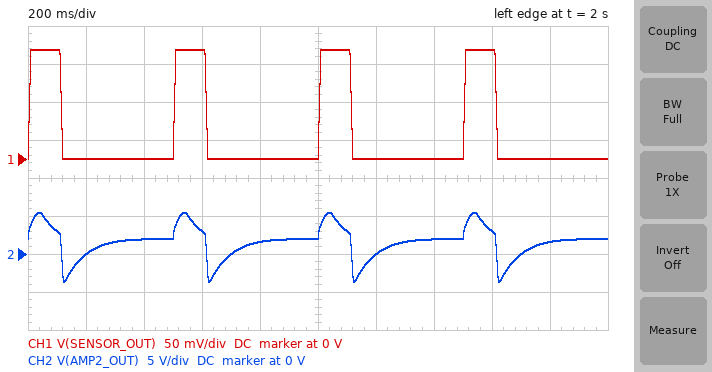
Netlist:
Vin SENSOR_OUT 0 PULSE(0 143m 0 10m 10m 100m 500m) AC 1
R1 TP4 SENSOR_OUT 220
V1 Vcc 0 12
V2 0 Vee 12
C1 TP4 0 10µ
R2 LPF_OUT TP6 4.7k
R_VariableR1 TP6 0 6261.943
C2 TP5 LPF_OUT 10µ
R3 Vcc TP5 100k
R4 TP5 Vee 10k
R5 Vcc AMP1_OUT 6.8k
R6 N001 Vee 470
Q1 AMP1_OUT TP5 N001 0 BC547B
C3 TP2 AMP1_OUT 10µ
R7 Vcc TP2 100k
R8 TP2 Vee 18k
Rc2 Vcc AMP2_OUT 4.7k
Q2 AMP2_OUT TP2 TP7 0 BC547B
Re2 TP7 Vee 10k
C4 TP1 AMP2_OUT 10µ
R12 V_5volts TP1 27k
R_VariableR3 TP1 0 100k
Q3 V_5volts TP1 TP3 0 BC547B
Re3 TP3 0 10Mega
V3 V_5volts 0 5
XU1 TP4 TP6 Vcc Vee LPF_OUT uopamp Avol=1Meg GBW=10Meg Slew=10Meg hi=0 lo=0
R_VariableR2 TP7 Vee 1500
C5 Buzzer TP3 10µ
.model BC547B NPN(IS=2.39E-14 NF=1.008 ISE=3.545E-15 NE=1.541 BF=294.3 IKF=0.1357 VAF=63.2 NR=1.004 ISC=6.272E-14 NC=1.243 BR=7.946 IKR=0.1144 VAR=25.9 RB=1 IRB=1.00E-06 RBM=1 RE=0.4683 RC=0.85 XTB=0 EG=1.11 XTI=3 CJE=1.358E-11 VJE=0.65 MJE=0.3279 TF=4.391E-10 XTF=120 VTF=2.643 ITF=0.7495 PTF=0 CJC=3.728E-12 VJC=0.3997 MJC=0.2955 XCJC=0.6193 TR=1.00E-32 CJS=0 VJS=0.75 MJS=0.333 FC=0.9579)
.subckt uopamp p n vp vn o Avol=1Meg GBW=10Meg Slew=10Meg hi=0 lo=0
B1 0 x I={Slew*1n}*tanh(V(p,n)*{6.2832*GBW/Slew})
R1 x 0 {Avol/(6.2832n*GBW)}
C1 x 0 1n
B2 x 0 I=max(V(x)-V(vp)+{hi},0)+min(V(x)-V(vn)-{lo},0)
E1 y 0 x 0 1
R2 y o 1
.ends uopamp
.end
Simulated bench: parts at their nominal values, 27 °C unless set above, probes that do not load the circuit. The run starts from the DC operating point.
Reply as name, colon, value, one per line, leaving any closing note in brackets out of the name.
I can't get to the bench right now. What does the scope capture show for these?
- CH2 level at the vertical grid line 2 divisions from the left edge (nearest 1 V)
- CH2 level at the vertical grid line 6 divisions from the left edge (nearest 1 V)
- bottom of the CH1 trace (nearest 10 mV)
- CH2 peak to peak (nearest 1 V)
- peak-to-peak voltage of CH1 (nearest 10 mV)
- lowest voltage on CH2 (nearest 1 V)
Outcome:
CH2 level at the vertical grid line 2 divisions from the left edge: 2 V
CH2 level at the vertical grid line 6 divisions from the left edge: 0 V
bottom of the CH1 trace: 0 V
CH2 peak to peak: 9 V
peak-to-peak voltage of CH1: 140 mV
lowest voltage on CH2: -4 V
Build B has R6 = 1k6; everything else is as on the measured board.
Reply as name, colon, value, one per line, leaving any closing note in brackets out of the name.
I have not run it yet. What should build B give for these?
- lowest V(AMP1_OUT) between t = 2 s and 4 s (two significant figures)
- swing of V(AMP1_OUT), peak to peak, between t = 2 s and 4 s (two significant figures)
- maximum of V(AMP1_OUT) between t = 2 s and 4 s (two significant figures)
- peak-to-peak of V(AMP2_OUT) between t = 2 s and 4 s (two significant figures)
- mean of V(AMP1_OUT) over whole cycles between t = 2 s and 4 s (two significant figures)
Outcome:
lowest V(AMP1_OUT) between t = 2 s and 4 s: 4.9 V
swing of V(AMP1_OUT), peak to peak, between t = 2 s and 4 s: 1.0 V
maximum of V(AMP1_OUT) between t = 2 s and 4 s: 5.9 V
peak-to-peak of V(AMP2_OUT) between t = 2 s and 4 s: 3.3 V
mean of V(AMP1_OUT) over whole cycles between t = 2 s and 4 s: 5.5 V
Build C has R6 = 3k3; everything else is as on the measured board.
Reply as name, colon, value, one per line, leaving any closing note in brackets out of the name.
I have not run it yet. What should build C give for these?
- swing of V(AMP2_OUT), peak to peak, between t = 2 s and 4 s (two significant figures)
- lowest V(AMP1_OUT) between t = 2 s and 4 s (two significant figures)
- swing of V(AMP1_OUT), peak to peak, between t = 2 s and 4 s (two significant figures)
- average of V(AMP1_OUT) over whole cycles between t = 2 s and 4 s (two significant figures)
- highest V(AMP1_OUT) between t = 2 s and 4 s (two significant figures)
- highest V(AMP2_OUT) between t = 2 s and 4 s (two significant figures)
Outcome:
swing of V(AMP2_OUT), peak to peak, between t = 2 s and 4 s: 1.7 V
lowest V(AMP1_OUT) between t = 2 s and 4 s: 8.5 V
swing of V(AMP1_OUT), peak to peak, between t = 2 s and 4 s: 500 mV
average of V(AMP1_OUT) over whole cycles between t = 2 s and 4 s: 8.8 V
highest V(AMP1_OUT) between t = 2 s and 4 s: 9.0 V
highest V(AMP2_OUT) between t = 2 s and 4 s: 2.5 V
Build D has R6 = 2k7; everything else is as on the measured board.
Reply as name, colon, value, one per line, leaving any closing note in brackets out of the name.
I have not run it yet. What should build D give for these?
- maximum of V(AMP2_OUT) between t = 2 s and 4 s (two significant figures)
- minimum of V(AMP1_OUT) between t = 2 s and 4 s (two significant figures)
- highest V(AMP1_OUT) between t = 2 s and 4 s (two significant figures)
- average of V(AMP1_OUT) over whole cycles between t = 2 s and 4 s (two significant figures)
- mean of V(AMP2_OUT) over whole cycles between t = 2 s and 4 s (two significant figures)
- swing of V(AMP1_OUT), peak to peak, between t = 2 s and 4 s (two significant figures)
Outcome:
maximum of V(AMP2_OUT) between t = 2 s and 4 s: 2.7 V
minimum of V(AMP1_OUT) between t = 2 s and 4 s: 7.7 V
highest V(AMP1_OUT) between t = 2 s and 4 s: 8.3 V
average of V(AMP1_OUT) over whole cycles between t = 2 s and 4 s: 8.1 V
mean of V(AMP2_OUT) over whole cycles between t = 2 s and 4 s: 1.6 V
swing of V(AMP1_OUT), peak to peak, between t = 2 s and 4 s: 610 mV
